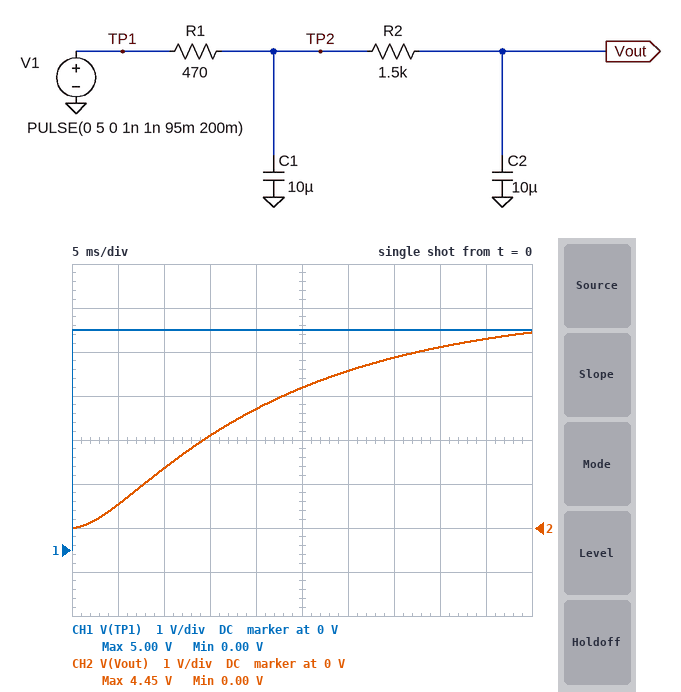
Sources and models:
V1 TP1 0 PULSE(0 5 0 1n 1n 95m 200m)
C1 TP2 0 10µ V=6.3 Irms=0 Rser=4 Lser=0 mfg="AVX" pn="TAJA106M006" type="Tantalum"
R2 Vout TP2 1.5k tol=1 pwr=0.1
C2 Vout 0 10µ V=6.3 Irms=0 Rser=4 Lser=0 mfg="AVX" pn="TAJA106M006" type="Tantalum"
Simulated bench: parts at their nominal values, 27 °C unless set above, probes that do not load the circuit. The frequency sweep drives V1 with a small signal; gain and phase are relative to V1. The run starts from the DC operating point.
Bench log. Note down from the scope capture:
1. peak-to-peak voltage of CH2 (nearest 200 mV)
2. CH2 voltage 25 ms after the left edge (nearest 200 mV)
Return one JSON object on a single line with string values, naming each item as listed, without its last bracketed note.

{"peak-to-peak voltage of CH2": "4.4 V", "CH2 voltage 25 ms after the left edge": "3.2 V"}
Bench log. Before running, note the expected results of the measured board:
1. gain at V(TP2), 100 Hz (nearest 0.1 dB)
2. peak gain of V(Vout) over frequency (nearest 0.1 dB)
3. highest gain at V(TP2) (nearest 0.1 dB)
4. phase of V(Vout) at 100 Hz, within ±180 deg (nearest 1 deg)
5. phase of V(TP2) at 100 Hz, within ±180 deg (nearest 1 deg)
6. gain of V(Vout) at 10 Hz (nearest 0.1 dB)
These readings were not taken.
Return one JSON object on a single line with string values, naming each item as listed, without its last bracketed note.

{"gain at V(TP2), 100 Hz": "-10.3 dB", "peak gain of V(Vout) over frequency": "0 dB", "highest gain at V(TP2)": "0 dB", "phase of V(Vout) at 100 Hz, within ±180 deg": "-148 deg", "phase of V(TP2) at 100 Hz, within ±180 deg": "-65 deg", "gain of V(Vout) at 10 Hz": "-4.6 dB"}
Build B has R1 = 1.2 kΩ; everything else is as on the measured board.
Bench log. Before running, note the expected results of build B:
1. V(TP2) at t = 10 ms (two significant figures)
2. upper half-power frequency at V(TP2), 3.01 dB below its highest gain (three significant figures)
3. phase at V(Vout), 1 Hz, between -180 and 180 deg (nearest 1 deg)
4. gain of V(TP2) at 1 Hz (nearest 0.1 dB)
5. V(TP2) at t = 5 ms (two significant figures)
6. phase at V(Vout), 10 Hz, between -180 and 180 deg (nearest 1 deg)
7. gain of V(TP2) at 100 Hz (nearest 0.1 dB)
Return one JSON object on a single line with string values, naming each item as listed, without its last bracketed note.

{"V(TP2) at t = 10 ms": "2.3 V", "upper half-power frequency at V(TP2), 3.01 dB below its highest gain": "5.79 Hz", "phase at V(Vout), 1 Hz, between -180 and 180 deg": "-14 deg", "gain of V(TP2) at 1 Hz": "-0.2 dB", "V(TP2) at t = 5 ms": "1.5 V", "phase at V(Vout), 10 Hz, between -180 and 180 deg": "-83 deg", "gain of V(TP2) at 100 Hz": "-17.9 dB"}
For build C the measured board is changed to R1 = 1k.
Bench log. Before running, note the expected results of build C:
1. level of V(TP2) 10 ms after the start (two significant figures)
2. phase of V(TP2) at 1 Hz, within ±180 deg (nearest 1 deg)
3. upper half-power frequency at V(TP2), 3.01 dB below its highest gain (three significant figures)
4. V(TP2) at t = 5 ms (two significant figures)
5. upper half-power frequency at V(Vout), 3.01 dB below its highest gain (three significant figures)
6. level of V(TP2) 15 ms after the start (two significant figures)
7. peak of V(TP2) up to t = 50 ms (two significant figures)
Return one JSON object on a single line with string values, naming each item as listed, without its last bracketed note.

{"level of V(TP2) 10 ms after the start": "2.6 V", "phase of V(TP2) at 1 Hz, within ±180 deg": "-7 deg", "upper half-power frequency at V(TP2), 3.01 dB below its highest gain": "6.98 Hz", "V(TP2) at t = 5 ms": "1.7 V", "upper half-power frequency at V(Vout), 3.01 dB below its highest gain": "5.16 Hz", "level of V(TP2) 15 ms after the start": "3.1 V", "peak of V(TP2) up to t = 50 ms": "4.4 V"}
